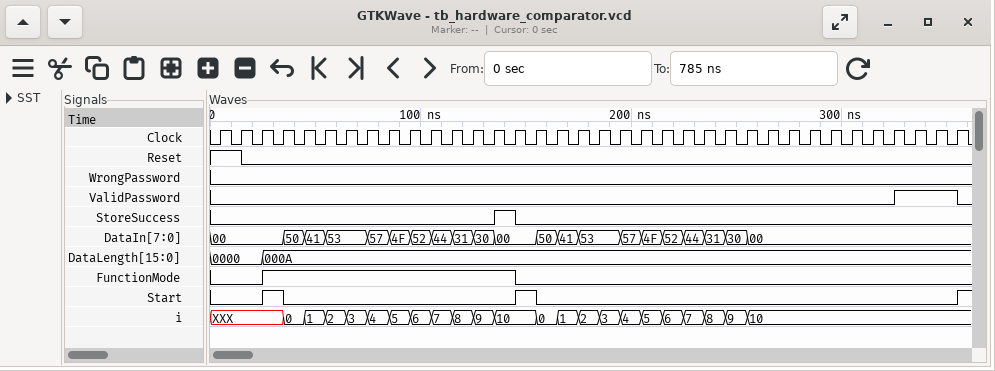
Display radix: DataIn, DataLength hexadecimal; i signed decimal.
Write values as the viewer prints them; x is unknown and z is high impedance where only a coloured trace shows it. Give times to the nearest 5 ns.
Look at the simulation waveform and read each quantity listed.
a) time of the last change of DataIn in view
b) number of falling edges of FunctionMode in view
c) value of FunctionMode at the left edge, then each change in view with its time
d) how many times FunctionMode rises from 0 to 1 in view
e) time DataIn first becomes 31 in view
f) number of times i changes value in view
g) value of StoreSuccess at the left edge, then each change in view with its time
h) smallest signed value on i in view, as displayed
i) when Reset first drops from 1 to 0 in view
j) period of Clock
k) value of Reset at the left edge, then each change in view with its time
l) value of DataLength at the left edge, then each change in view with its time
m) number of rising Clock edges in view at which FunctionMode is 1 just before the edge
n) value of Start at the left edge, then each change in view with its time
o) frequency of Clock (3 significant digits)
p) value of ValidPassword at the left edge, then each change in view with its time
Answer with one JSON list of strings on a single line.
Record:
["255 ns", "1", "0, 1 at 25 ns, 0 at 145 ns", "1", "115 ns", "22", "0, 1 at 135 ns, 0 at 145 ns", "0", "15 ns", "10 ns", "1, 0 at 15 ns", "0000, 000A at 25 ns", "12", "0, 1 at 25 ns, 0 at 35 ns, 1 at 145 ns, 0 at 155 ns, 1 at 355 ns", "100 MHz", "0, 1 at 325 ns, 0 at 355 ns"]
